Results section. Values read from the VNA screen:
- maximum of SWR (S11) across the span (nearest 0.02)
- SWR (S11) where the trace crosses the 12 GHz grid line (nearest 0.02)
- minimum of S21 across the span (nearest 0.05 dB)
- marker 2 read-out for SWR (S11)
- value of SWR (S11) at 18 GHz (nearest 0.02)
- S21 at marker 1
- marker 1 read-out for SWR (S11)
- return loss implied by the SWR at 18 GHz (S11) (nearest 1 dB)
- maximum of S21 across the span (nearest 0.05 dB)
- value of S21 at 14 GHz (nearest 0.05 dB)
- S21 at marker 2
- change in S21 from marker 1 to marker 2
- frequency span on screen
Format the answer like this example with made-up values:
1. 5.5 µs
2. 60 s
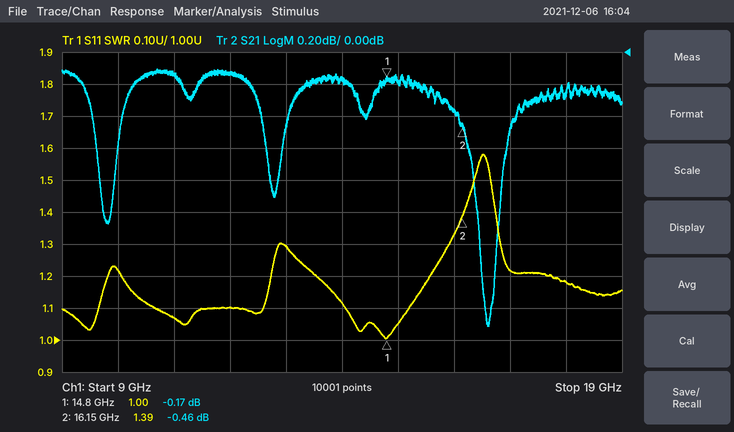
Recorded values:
1. 1.58
2. 1.10
3. -1.70 dB
4. 1.39
5. 1.18
6. -0.17 dB
7. 1.00
8. 22 dB
9. -0.10 dB
10. -0.15 dB
11. -0.46 dB
12. -0.29 dB
13. 10 GHz
